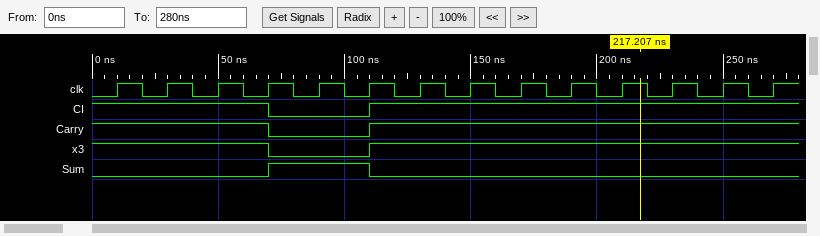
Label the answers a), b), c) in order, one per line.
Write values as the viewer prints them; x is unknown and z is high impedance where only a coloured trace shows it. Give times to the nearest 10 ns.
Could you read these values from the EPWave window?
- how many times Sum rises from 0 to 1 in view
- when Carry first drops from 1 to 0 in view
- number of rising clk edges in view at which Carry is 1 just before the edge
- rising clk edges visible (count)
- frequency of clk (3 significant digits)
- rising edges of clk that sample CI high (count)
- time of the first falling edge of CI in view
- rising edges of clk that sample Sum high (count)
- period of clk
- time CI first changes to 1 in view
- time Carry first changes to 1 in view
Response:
a) 1
b) 70 ns
c) 12
d) 14
e) 50.0 MHz
f) 12
g) 70 ns
h) 2
i) 20 ns
j) 110 ns
k) 110 ns
